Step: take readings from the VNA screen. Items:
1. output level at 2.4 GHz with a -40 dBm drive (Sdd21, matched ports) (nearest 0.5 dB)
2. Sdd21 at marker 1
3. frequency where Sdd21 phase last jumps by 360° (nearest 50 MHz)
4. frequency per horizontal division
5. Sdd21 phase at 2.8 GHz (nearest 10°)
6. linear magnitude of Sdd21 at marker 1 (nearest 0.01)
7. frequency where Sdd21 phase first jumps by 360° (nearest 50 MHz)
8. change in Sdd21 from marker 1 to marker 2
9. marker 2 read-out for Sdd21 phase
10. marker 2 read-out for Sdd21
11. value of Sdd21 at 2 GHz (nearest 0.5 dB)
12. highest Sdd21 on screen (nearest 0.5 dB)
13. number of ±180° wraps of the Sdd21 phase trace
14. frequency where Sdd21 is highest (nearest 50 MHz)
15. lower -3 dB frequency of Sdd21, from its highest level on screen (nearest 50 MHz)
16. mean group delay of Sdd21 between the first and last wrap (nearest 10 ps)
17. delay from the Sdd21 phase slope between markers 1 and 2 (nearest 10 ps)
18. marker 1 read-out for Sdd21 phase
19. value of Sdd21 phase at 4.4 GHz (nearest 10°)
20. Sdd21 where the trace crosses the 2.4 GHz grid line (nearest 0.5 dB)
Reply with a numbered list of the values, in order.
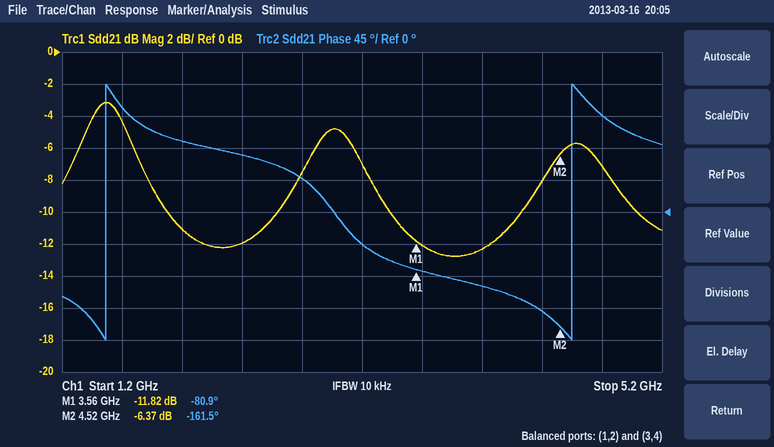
1. -52.0 dBm
2. -11.82 dB
3. 4.60 GHz
4. 400 MHz
5. 50°
6. 0.26
7. 1.50 GHz
8. 5.45 dB
9. -161.5°
10. -6.37 dB
11. -11.0 dB
12. -3.0 dB
13. 2
14. 1.50 GHz
15. 1.30 GHz
16. 320 ps
17. 230 ps
18. -80.9°
19. -140°
20. -12.0 dB
